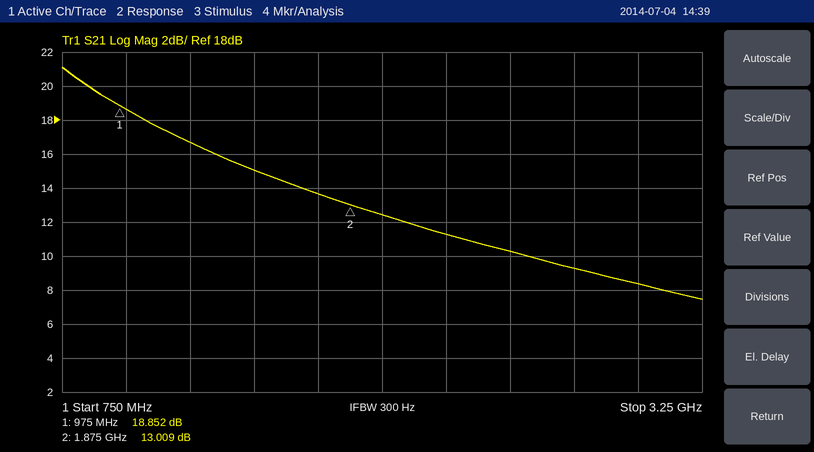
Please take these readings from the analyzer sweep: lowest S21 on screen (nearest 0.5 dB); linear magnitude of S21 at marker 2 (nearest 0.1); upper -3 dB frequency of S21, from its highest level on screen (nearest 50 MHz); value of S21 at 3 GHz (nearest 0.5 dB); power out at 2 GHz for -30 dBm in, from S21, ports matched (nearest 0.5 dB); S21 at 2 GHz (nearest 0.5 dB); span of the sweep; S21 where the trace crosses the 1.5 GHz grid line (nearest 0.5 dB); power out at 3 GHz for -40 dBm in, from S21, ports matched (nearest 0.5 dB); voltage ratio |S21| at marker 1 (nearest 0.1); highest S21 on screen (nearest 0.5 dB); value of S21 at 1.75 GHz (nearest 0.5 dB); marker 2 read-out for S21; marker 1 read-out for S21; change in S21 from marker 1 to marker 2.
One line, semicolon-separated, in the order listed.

7.5 dB; 4.5; 1.05 GHz; 8.5 dB; -17.5 dBm; 12.5 dB; 2.5 GHz; 15.0 dB; -31.5 dBm; 8.8; 21.0 dB; 13.5 dB; 13.009 dB; 18.852 dB; -5.843 dB
